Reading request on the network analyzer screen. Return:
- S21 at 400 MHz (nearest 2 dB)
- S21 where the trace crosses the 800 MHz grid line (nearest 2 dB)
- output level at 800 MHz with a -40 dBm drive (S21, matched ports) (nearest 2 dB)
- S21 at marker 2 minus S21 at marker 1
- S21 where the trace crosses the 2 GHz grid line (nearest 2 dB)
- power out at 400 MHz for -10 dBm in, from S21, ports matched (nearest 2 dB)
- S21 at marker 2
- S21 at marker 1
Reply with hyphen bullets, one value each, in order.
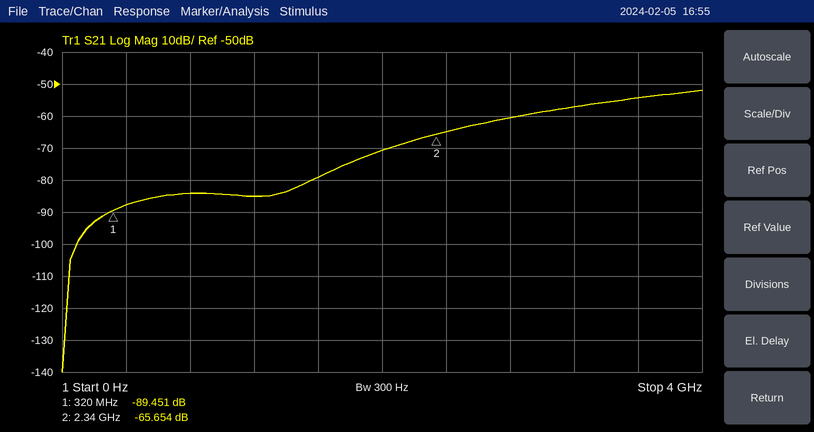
- -88 dB
- -84 dB
- -124 dBm
- 23.797 dB
- -70 dB
- -98 dBm
- -65.654 dB
- -89.451 dB
